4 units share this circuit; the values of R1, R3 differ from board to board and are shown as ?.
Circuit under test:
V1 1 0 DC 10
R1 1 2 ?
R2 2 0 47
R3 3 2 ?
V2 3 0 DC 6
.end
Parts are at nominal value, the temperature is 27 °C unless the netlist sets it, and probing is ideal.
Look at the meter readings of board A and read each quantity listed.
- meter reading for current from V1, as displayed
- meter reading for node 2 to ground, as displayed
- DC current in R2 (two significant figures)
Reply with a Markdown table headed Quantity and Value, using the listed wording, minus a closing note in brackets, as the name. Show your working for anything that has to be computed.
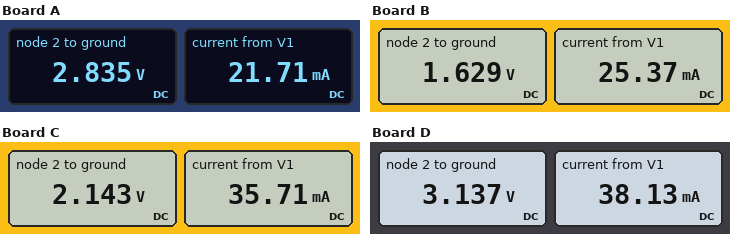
| Quantity | Value |
|---|---|
| meter reading for current from V1, as displayed | 21.71 mA |
| meter reading for node 2 to ground, as displayed | 2.835 V |
| DC current in R2 | (2.835 V) / 47 Ω = 60 mA |
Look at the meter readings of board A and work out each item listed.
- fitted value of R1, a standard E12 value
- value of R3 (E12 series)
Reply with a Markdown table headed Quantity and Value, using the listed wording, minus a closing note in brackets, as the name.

| Quantity | Value |
|---|---|
| fitted value of R1, a standard E12 value | 330 Ω |
| value of R3 | 82 Ω |
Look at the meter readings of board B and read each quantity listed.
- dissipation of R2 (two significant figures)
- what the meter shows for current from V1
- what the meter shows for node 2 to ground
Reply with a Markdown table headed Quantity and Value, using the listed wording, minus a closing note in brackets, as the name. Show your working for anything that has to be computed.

| Quantity | Value |
|---|---|
| dissipation of R2 | (1.629 V)^2 / 47 Ω = 56 mW |
| what the meter shows for current from V1 | 25.37 mA |
| what the meter shows for node 2 to ground | 1.629 V |
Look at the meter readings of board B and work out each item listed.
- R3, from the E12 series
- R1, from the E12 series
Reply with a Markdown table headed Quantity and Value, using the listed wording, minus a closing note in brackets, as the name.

| Quantity | Value |
|---|---|
| R3, from the E12 series | 470 Ω |
| R1, from the E12 series | 330 Ω |
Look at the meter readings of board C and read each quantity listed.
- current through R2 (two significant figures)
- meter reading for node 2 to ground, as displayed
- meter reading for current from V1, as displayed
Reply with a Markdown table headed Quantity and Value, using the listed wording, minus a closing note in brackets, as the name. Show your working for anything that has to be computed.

| Quantity | Value |
|---|---|
| current through R2 | (2.143 V) / 47 Ω = 46 mA |
| meter reading for node 2 to ground, as displayed | 2.143 V |
| meter reading for current from V1, as displayed | 35.71 mA |
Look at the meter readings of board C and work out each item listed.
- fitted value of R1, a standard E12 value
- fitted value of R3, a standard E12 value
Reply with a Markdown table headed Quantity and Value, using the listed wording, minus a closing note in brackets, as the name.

| Quantity | Value |
|---|---|
| fitted value of R1, a standard E12 value | 220 Ω |
| fitted value of R3, a standard E12 value | 390 Ω |
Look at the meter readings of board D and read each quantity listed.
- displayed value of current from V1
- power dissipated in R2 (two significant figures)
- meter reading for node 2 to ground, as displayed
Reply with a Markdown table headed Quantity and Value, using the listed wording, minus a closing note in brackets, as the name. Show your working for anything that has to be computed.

| Quantity | Value |
|---|---|
| displayed value of current from V1 | 38.13 mA |
| power dissipated in R2 | (3.137 V)^2 / 47 Ω = 210 mW |
| meter reading for node 2 to ground, as displayed | 3.137 V |
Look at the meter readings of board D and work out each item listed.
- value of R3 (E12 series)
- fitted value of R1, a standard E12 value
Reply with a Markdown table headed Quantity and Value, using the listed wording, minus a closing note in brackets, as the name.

| Quantity | Value |
|---|---|
| value of R3 | 100 Ω |
| fitted value of R1, a standard E12 value | 180 Ω |
